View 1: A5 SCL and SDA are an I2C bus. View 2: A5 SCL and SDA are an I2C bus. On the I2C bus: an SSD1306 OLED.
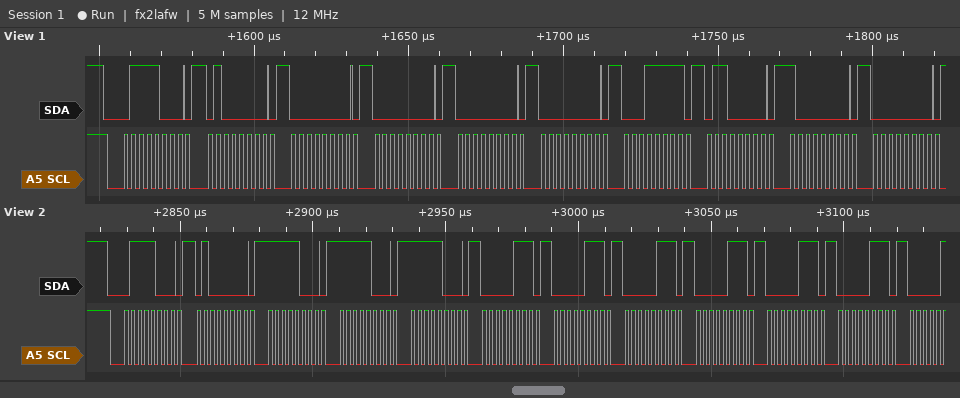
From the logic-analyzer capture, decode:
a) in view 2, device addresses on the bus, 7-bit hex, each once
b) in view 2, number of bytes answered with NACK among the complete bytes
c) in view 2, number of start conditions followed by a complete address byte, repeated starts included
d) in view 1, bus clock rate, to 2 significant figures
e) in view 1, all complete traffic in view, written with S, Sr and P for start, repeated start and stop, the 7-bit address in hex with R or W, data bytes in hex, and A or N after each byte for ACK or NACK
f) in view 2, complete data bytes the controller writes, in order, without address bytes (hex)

0x3C
0
1
400 kHz
S 3CW A 40 A 00 A 00 A 00 A 00 A 1F A 60 A 80 A 00 A
40 F8 F8 F8 07 07 07 07 07 07
